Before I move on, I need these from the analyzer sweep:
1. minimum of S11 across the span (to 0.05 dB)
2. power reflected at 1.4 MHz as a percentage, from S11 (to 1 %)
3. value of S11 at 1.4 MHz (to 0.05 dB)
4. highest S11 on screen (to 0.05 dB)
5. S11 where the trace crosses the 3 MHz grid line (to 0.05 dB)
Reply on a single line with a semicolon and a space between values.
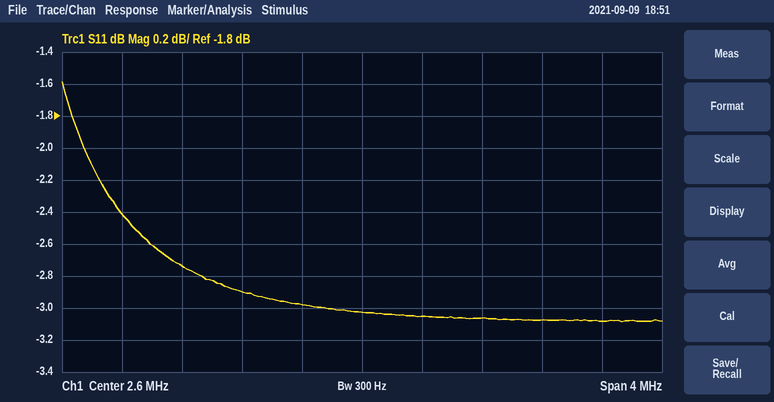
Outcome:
-3.10 dB; 53 %; -2.75 dB; -1.60 dB; -3.05 dB
